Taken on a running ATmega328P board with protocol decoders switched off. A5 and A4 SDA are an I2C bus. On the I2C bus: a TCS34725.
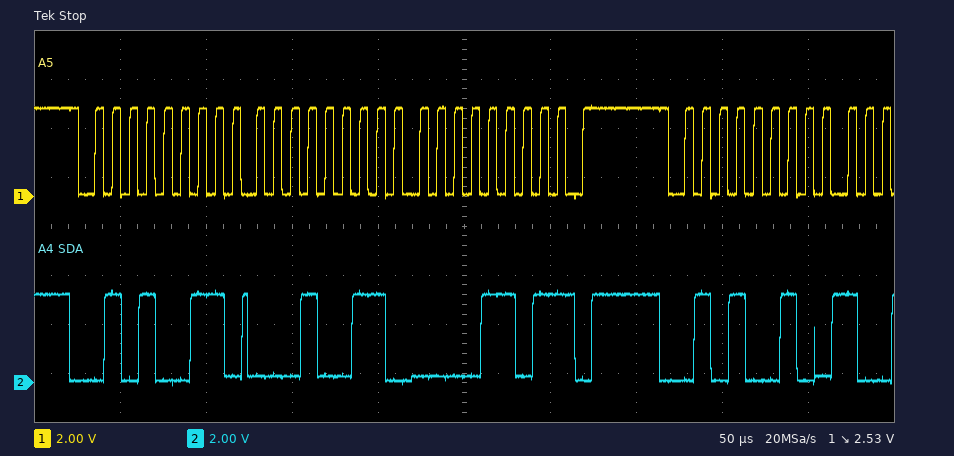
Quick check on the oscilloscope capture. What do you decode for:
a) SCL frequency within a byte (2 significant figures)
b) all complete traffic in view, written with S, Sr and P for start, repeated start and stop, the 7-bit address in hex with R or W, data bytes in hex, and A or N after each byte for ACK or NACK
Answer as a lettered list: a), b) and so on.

a) 100 kHz
b) S 29R A 13 A 0D N P S 29W A
